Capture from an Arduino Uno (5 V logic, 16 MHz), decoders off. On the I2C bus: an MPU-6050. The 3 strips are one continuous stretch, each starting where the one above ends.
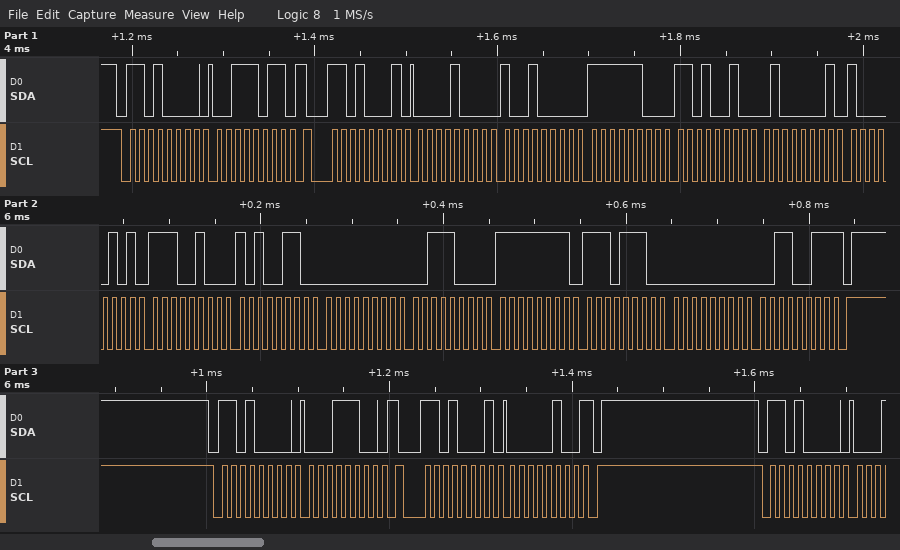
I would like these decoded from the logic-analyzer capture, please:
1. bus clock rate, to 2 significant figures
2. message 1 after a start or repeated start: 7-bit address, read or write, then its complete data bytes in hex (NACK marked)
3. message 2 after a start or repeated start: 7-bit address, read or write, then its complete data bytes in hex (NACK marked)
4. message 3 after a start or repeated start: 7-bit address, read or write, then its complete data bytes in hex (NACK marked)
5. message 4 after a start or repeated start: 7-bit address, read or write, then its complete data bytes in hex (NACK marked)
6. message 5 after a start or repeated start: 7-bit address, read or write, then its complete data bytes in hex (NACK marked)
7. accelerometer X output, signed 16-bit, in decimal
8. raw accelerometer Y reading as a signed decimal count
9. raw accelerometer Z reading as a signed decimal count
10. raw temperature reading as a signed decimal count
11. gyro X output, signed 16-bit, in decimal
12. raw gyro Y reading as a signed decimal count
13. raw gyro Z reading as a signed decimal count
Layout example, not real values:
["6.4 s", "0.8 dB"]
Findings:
["100 kHz", "0x68 write: 3B", "0x68 read: 08 90 FC D2 41 85 E4 A6 00 38 FF EE 00 33 NACK", "0x68 write: 1C", "0x68 read: 04 NACK", "0x68 write", "2192", "-814", "16773", "-7002", "56", "-18", "51"]
